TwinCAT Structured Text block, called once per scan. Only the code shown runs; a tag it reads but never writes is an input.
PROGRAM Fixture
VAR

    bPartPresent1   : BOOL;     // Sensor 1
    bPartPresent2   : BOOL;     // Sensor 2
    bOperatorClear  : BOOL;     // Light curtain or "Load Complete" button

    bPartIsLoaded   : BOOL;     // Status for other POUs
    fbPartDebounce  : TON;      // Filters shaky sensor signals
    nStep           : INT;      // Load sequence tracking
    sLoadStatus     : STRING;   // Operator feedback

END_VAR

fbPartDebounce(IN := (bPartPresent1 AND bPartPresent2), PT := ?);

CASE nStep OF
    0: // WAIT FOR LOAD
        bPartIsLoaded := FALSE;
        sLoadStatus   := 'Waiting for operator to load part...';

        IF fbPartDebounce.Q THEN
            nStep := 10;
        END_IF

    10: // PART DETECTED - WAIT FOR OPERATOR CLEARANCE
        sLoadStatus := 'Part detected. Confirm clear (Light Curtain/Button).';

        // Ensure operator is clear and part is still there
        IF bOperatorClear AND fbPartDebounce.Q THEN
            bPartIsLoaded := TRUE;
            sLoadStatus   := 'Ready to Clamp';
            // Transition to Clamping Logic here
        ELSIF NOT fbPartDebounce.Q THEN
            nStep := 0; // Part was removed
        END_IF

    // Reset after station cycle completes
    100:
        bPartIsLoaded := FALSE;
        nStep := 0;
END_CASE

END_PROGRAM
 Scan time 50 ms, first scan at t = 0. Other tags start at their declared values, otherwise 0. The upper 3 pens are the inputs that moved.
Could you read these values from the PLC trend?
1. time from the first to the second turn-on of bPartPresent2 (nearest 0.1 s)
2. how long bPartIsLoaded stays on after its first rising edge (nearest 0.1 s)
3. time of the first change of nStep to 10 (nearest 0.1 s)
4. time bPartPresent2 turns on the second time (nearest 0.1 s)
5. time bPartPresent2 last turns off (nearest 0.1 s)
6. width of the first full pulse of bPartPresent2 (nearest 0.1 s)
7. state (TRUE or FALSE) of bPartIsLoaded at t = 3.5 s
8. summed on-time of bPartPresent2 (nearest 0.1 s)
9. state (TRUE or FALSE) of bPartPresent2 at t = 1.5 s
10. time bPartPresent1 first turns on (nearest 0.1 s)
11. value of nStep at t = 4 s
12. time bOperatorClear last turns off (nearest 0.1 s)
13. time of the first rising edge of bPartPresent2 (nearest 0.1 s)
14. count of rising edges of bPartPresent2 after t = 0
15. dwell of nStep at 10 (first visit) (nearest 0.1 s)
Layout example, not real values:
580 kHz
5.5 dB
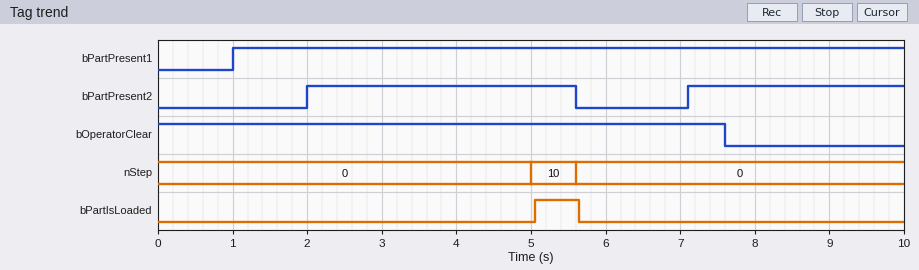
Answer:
5.1 s
0.6 s
5.0 s
7.1 s
5.6 s
3.6 s
FALSE
6.5 s
FALSE
1.0 s
0
7.6 s
2.0 s
2
0.6 s
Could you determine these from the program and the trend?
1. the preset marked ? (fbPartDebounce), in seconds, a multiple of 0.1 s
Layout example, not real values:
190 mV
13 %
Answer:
3.0 s
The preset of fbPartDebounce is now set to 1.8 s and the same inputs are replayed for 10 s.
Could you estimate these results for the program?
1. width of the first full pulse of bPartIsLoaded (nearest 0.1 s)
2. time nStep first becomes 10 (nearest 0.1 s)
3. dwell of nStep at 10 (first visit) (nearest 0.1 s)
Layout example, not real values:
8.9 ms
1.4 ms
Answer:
1.8 s
3.8 s
1.8 s
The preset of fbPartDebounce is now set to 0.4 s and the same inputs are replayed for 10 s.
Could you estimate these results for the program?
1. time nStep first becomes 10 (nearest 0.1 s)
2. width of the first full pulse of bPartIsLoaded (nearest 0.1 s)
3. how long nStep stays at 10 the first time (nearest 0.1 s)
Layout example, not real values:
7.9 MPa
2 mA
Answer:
2.4 s
3.2 s
3.2 s
